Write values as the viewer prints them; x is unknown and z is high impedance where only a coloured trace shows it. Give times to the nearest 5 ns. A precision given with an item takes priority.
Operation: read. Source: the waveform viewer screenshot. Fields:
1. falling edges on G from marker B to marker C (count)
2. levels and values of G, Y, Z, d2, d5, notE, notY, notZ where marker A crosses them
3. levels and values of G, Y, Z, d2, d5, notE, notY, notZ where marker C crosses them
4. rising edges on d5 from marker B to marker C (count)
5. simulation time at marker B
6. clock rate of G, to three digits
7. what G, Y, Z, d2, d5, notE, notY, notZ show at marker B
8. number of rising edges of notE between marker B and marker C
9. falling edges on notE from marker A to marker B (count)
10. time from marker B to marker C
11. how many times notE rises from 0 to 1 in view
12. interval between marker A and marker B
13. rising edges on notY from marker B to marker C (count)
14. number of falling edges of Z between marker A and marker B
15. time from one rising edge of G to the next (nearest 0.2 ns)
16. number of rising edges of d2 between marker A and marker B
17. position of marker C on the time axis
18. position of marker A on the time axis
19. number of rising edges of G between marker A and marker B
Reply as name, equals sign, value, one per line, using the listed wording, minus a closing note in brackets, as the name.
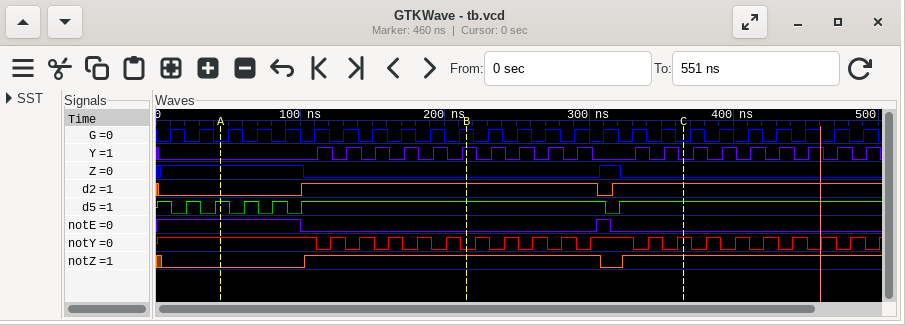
falling edges on G from marker B to marker C = 8
levels and values of G, Y, Z, d2, d5, notE, notY, notZ where marker A crosses them = G=0, Y=0, Z=1, d2=0, d5=1, notE=1, notY=1, notZ=0
levels and values of G, Y, Z, d2, d5, notE, notY, notZ where marker C crosses them = G=0, Y=0, Z=0, d2=1, d5=1, notE=0, notY=1, notZ=1
rising edges on d5 from marker B to marker C = 1
simulation time at marker B = 215 ns
clock rate of G, to three digits = 50.0 MHz
what G, Y, Z, d2, d5, notE, notY, notZ show at marker B = G=1, Y=1, Z=0, d2=1, d5=1, notE=0, notY=0, notZ=1
number of rising edges of notE between marker B and marker C = 1
falling edges on notE from marker A to marker B = 1
time from marker B to marker C = 150 ns
how many times notE rises from 0 to 1 in view = 1
interval between marker A and marker B = 170 ns
rising edges on notY from marker B to marker C = 7
number of falling edges of Z between marker A and marker B = 1
time from one rising edge of G to the next = 20 ns
number of rising edges of d2 between marker A and marker B = 1
position of marker C on the time axis = 365 ns
position of marker A on the time axis = 45 ns
number of rising edges of G between marker A and marker B = 9
